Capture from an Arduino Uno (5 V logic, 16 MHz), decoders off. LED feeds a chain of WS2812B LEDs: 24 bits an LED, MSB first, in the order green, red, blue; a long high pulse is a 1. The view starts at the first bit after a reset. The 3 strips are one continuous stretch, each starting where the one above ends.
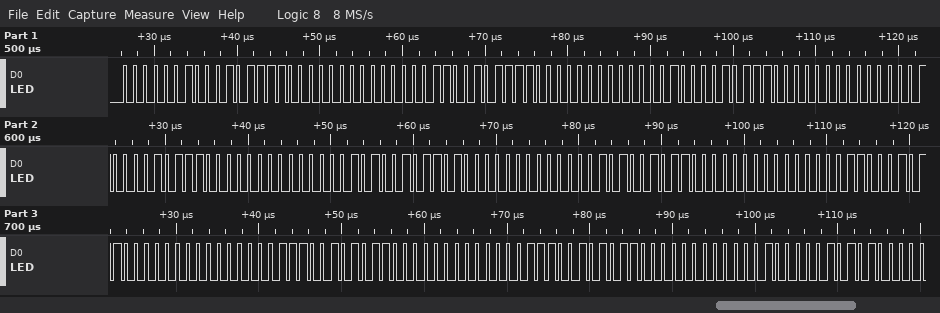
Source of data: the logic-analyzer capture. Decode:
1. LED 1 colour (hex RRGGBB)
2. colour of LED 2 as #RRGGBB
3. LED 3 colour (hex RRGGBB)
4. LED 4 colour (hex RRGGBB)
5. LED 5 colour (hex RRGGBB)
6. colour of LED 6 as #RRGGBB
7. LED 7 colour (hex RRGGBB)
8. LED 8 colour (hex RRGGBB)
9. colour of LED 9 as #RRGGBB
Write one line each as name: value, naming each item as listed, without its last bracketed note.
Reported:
LED 1 colour: #2F0200
colour of LED 2 as #RRGGBB: #2F0300
LED 3 colour: #2E0400
LED 4 colour: #2E0400
LED 5 colour: #2D0500
colour of LED 6 as #RRGGBB: #2C0500
LED 7 colour: #2C0600
LED 8 colour: #2B0700
colour of LED 9 as #RRGGBB: #2B0700
